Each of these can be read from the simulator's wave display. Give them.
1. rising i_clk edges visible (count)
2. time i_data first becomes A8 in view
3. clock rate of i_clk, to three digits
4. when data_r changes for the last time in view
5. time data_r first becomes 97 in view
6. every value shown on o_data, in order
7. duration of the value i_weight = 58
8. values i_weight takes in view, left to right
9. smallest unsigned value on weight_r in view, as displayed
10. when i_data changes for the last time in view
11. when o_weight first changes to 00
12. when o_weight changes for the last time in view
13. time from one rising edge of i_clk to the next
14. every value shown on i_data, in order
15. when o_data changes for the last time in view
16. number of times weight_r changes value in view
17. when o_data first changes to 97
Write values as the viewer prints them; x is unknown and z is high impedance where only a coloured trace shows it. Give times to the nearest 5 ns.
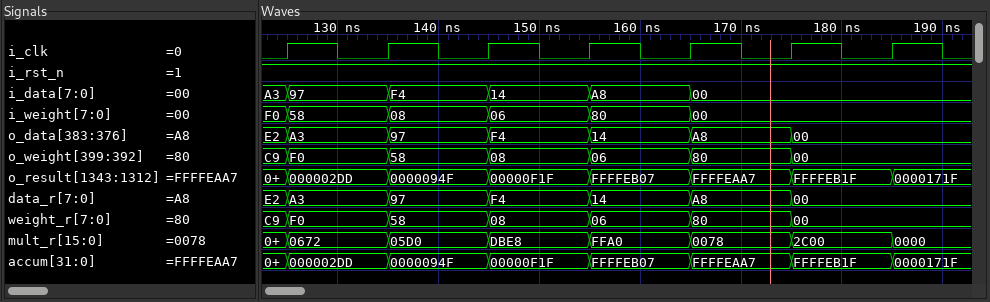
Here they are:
7
155 ns
100 MHz
175 ns
135 ns
E2, A3, 97, F4, 14, A8, 00
10 ns
F0, 58, 08, 06, 80, 00
00
165 ns
175 ns
175 ns
10 ns
A3, 97, F4, 14, A8, 00
175 ns
6
135 ns
